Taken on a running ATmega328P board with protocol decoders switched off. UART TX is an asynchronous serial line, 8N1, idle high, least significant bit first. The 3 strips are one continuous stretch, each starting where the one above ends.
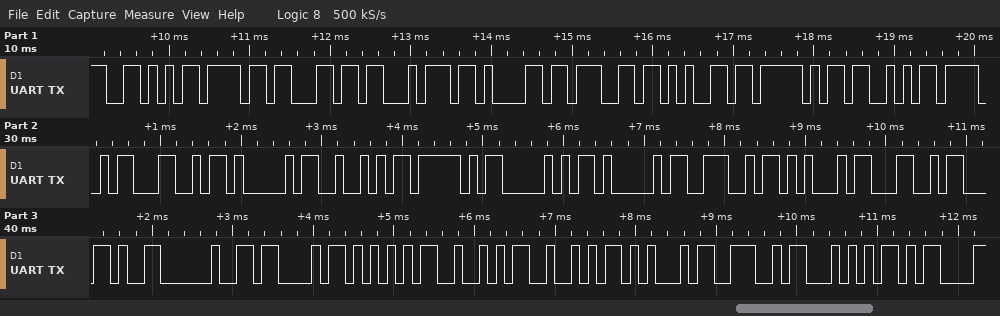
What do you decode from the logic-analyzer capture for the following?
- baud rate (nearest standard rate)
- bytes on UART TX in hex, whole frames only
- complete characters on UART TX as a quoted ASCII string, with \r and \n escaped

9600 baud
56 6F 6C 74 61 67 65 5F 53 4F 4C 41 52 5F 50 41 4E 45 4C 2C 20 43 55 52 52 45 4E 54 0D
"Voltage_SOLAR_PANEL, CURRENT\r"
